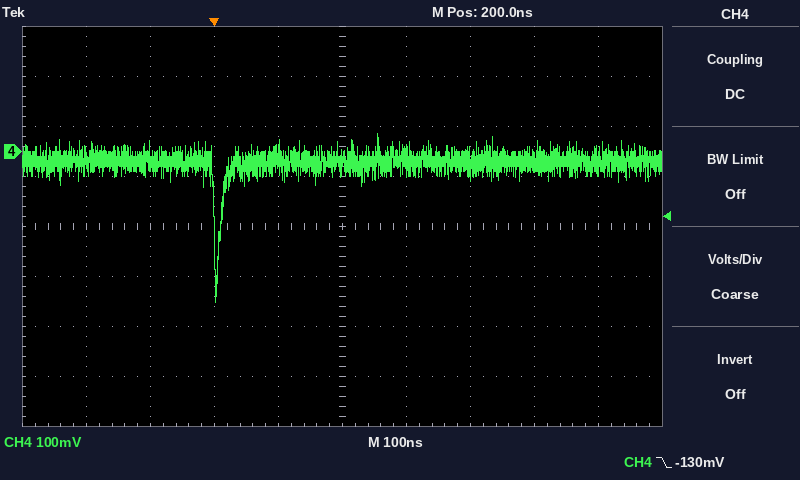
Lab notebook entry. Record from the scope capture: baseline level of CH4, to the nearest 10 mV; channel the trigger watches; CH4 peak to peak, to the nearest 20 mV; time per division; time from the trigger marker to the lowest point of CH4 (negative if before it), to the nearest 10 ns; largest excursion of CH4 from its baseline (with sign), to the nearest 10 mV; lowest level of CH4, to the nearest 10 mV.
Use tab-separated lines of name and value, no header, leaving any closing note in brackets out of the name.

baseline level of CH4, to the nearest 10 mV	-20 mV
channel the trigger watches	CH4
CH4 peak to peak, to the nearest 20 mV	340 mV
time per division	100 ns
time from the trigger marker to the lowest point of CH4 (negative if before it), to the nearest 10 ns	0 ns
largest excursion of CH4 from its baseline (with sign), to the nearest 10 mV	-280 mV
lowest level of CH4, to the nearest 10 mV	-300 mV
